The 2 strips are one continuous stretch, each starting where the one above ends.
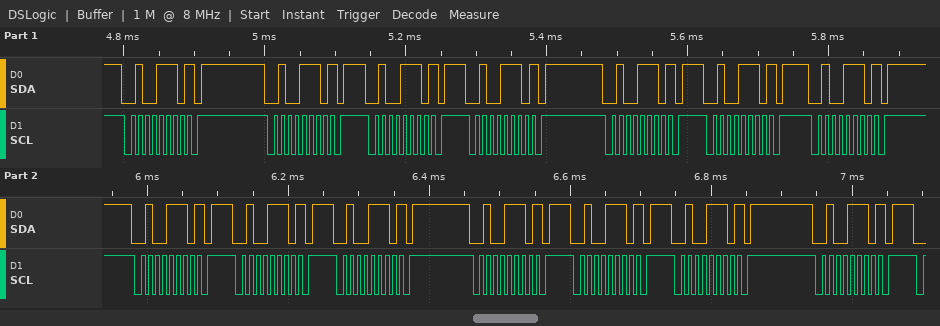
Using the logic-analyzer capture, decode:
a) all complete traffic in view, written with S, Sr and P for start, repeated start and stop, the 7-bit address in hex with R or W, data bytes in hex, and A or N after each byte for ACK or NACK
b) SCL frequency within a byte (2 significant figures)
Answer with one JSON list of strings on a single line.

["S 27W N P S 27W N P S 27W N P S 27W N P S 27W N P S 27W N P S 27W N P S 27W N P S 27W N P S 27W N P S 27W N P S 27W N P S 27W N P S 27W N P", "100 kHz"]
